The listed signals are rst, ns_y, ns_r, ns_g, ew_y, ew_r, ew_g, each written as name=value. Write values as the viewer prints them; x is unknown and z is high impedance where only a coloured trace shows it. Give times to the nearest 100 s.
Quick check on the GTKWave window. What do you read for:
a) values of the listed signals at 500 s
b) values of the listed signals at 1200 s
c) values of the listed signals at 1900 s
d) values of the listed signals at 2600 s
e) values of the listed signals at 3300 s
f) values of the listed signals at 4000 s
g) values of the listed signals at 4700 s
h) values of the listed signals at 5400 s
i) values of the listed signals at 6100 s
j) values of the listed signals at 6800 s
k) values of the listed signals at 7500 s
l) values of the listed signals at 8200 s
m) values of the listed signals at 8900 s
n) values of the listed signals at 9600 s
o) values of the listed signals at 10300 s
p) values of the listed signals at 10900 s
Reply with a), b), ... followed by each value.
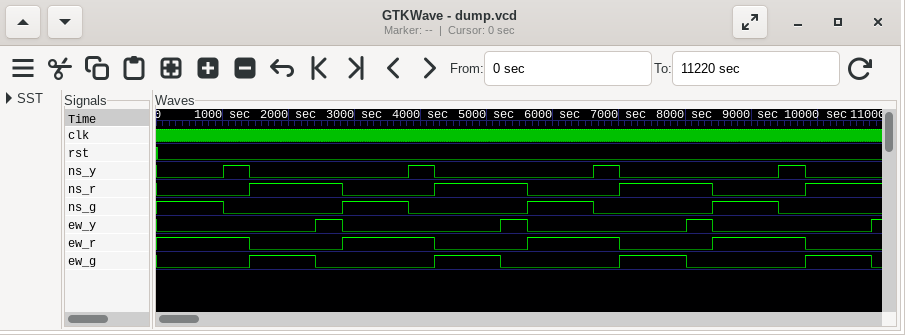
a) rst=0, ns_y=0, ns_r=0, ns_g=1, ew_y=0, ew_r=1, ew_g=0
b) rst=0, ns_y=1, ns_r=0, ns_g=0, ew_y=0, ew_r=1, ew_g=0
c) rst=0, ns_y=0, ns_r=1, ns_g=0, ew_y=0, ew_r=0, ew_g=1
d) rst=0, ns_y=0, ns_r=1, ns_g=0, ew_y=1, ew_r=0, ew_g=0
e) rst=0, ns_y=0, ns_r=0, ns_g=1, ew_y=0, ew_r=1, ew_g=0
f) rst=0, ns_y=1, ns_r=0, ns_g=0, ew_y=0, ew_r=1, ew_g=0
g) rst=0, ns_y=0, ns_r=1, ns_g=0, ew_y=0, ew_r=0, ew_g=1
h) rst=0, ns_y=0, ns_r=1, ns_g=0, ew_y=1, ew_r=0, ew_g=0
i) rst=0, ns_y=0, ns_r=0, ns_g=1, ew_y=0, ew_r=1, ew_g=0
j) rst=0, ns_y=1, ns_r=0, ns_g=0, ew_y=0, ew_r=1, ew_g=0
k) rst=0, ns_y=0, ns_r=1, ns_g=0, ew_y=0, ew_r=0, ew_g=1
l) rst=0, ns_y=0, ns_r=1, ns_g=0, ew_y=1, ew_r=0, ew_g=0
m) rst=0, ns_y=0, ns_r=0, ns_g=1, ew_y=0, ew_r=1, ew_g=0
n) rst=0, ns_y=1, ns_r=0, ns_g=0, ew_y=0, ew_r=1, ew_g=0
o) rst=0, ns_y=0, ns_r=1, ns_g=0, ew_y=0, ew_r=0, ew_g=1
p) rst=0, ns_y=0, ns_r=1, ns_g=0, ew_y=1, ew_r=0, ew_g=0
